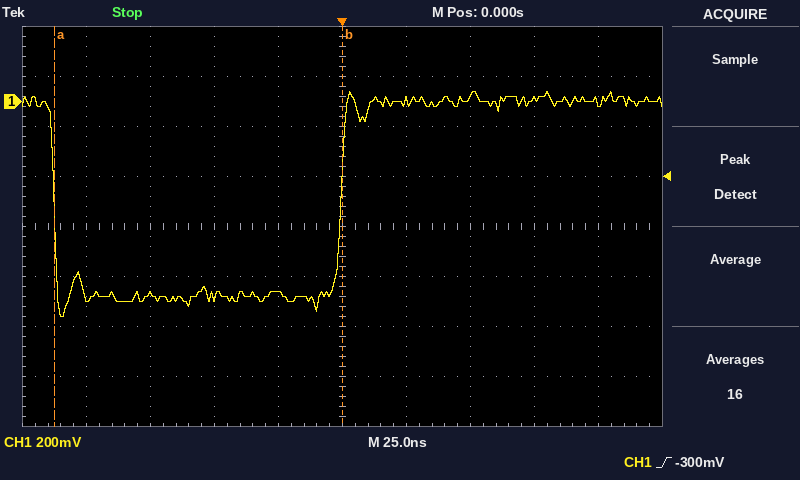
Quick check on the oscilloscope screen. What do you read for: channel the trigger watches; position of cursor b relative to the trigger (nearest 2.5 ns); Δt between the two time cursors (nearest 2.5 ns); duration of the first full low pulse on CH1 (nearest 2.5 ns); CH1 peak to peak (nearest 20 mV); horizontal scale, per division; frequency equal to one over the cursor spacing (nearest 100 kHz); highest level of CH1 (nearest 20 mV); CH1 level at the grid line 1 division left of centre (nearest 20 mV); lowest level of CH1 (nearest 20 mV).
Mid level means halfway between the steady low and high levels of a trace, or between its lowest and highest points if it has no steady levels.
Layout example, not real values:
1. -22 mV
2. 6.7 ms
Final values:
1. CH1
2. 0.0 ns
3. 112.5 ns
4. 112.5 ns
5. 900 mV
6. 25 ns
7. 8.9 MHz
8. 40 mV
9. -760 mV
10. -860 mV
